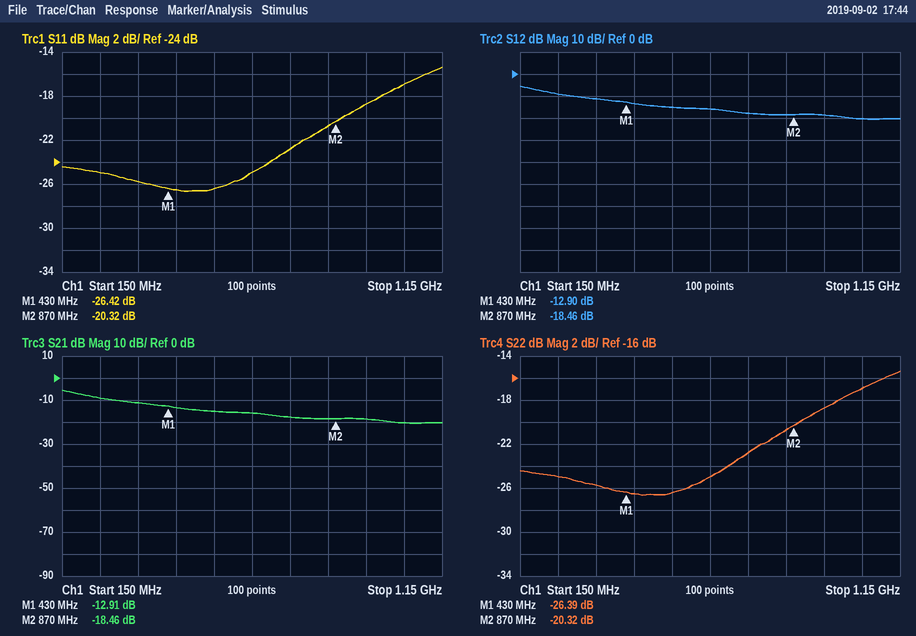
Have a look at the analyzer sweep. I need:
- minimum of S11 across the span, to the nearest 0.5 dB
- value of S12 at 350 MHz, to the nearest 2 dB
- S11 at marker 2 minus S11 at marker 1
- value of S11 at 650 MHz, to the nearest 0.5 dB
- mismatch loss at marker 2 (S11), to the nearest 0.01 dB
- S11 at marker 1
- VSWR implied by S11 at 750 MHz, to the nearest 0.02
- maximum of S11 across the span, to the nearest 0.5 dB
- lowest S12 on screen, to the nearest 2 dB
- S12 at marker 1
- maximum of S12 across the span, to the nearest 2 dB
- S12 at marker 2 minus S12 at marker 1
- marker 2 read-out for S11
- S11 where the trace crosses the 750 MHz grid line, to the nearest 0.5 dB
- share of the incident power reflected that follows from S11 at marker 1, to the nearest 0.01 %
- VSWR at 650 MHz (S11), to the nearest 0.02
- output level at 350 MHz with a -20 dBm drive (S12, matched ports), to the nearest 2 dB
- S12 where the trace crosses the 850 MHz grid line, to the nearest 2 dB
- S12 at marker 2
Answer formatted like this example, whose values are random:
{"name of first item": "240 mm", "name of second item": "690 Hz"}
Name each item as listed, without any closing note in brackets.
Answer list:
{"minimum of S11 across the span, to the nearest 0.5 dB": "-26.5 dB", "value of S12 at 350 MHz, to the nearest 2 dB": "-12 dB", "S11 at marker 2 minus S11 at marker 1": "6.10 dB", "value of S11 at 650 MHz, to the nearest 0.5 dB": "-25.0 dB", "mismatch loss at marker 2 (S11), to the nearest 0.01 dB": "0.04 dB", "S11 at marker 1": "-26.42 dB", "VSWR implied by S11 at 750 MHz, to the nearest 0.02": "1.16", "maximum of S11 across the span, to the nearest 0.5 dB": "-15.5 dB", "lowest S12 on screen, to the nearest 2 dB": "-20 dB", "S12 at marker 1": "-12.90 dB", "maximum of S12 across the span, to the nearest 2 dB": "-6 dB", "S12 at marker 2 minus S12 at marker 1": "-5.56 dB", "marker 2 read-out for S11": "-20.32 dB", "S11 where the trace crosses the 750 MHz grid line, to the nearest 0.5 dB": "-23.0 dB", "share of the incident power reflected that follows from S11 at marker 1, to the nearest 0.01 %": "0.23 %", "VSWR at 650 MHz (S11), to the nearest 0.02": "1.12", "output level at 350 MHz with a -20 dBm drive (S12, matched ports), to the nearest 2 dB": "-32 dBm", "S12 where the trace crosses the 850 MHz grid line, to the nearest 2 dB": "-18 dB", "S12 at marker 2": "-18.46 dB"}
